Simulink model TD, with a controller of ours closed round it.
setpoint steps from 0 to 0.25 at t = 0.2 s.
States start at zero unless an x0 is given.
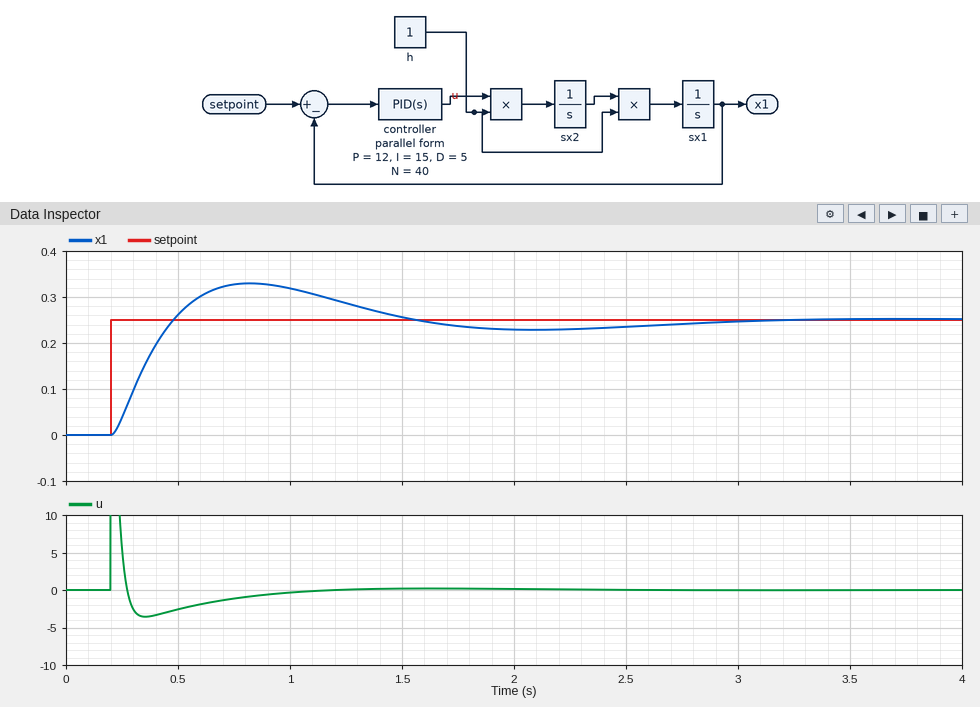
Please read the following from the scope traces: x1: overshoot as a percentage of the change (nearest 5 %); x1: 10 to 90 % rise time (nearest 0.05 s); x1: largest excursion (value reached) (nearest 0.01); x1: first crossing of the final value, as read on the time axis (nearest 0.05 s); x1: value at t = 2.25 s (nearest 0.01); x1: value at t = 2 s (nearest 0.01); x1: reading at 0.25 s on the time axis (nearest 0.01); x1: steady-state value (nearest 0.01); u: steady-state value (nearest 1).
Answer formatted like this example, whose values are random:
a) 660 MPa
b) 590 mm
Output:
a) 30 %
b) 0.20 s
c) 0.33
d) 0.50 s
e) 0.23
f) 0.23
g) 0.04
h) 0.25
i) 0
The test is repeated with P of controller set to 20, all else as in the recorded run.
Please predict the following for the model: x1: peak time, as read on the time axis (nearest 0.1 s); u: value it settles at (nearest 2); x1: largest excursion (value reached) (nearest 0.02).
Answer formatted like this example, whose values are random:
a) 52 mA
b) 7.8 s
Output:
a) 0.7 s
b) 0
c) 0.34
